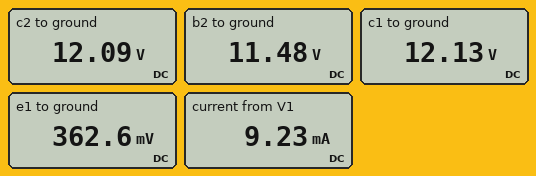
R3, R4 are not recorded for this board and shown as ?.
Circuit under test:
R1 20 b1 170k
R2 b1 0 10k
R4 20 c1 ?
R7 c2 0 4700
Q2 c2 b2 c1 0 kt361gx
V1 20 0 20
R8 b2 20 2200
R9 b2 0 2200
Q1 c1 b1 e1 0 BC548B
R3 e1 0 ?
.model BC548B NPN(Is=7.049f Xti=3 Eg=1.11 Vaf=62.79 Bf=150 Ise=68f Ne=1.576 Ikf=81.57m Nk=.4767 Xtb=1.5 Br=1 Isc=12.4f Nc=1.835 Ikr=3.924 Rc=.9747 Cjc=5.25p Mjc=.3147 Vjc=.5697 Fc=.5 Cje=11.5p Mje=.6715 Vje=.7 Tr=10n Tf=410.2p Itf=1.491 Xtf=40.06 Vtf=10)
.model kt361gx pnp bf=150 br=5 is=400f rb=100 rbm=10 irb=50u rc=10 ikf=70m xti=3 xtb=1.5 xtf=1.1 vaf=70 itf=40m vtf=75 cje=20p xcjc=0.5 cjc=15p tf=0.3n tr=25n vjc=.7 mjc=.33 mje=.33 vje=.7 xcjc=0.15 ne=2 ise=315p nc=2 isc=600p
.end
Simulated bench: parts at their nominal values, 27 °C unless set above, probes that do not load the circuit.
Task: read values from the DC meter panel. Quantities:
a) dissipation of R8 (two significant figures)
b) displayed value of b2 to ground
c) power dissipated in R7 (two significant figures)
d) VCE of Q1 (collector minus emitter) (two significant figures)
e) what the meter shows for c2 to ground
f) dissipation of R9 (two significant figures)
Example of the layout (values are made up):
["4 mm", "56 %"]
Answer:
["33 mW", "11.48 V", "31 mW", "12 V", "12.09 V", "60 mW"]
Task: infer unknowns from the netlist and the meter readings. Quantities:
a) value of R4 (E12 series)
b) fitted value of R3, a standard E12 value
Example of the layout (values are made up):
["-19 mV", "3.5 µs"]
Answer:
["1.5 kΩ", "270 Ω"]
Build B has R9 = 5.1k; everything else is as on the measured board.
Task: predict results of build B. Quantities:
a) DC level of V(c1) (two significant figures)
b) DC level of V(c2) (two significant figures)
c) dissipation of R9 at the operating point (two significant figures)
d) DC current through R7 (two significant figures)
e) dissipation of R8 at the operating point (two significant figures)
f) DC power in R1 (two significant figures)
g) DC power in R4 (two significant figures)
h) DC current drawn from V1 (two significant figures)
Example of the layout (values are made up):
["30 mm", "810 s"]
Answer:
["15 V", "10 V", "39 mW", "2.2 mA", "16 mW", "2.1 mW", "19 mW", "6.4 mA"]
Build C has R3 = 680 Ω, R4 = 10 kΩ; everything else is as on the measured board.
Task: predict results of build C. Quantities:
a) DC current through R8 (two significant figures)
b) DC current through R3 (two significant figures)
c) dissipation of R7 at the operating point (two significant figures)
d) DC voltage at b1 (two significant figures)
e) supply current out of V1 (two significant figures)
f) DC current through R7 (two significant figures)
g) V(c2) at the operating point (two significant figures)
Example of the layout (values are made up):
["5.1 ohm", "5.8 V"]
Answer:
["4.5 mA", "620 µA", "470 µW", "1.1 V", "5.6 mA", "320 µA", "1.5 V"]
